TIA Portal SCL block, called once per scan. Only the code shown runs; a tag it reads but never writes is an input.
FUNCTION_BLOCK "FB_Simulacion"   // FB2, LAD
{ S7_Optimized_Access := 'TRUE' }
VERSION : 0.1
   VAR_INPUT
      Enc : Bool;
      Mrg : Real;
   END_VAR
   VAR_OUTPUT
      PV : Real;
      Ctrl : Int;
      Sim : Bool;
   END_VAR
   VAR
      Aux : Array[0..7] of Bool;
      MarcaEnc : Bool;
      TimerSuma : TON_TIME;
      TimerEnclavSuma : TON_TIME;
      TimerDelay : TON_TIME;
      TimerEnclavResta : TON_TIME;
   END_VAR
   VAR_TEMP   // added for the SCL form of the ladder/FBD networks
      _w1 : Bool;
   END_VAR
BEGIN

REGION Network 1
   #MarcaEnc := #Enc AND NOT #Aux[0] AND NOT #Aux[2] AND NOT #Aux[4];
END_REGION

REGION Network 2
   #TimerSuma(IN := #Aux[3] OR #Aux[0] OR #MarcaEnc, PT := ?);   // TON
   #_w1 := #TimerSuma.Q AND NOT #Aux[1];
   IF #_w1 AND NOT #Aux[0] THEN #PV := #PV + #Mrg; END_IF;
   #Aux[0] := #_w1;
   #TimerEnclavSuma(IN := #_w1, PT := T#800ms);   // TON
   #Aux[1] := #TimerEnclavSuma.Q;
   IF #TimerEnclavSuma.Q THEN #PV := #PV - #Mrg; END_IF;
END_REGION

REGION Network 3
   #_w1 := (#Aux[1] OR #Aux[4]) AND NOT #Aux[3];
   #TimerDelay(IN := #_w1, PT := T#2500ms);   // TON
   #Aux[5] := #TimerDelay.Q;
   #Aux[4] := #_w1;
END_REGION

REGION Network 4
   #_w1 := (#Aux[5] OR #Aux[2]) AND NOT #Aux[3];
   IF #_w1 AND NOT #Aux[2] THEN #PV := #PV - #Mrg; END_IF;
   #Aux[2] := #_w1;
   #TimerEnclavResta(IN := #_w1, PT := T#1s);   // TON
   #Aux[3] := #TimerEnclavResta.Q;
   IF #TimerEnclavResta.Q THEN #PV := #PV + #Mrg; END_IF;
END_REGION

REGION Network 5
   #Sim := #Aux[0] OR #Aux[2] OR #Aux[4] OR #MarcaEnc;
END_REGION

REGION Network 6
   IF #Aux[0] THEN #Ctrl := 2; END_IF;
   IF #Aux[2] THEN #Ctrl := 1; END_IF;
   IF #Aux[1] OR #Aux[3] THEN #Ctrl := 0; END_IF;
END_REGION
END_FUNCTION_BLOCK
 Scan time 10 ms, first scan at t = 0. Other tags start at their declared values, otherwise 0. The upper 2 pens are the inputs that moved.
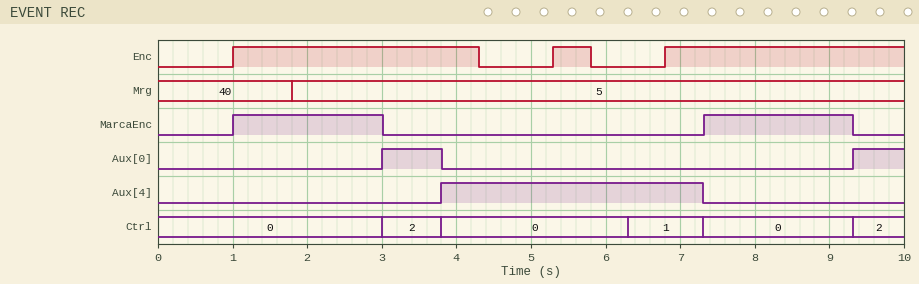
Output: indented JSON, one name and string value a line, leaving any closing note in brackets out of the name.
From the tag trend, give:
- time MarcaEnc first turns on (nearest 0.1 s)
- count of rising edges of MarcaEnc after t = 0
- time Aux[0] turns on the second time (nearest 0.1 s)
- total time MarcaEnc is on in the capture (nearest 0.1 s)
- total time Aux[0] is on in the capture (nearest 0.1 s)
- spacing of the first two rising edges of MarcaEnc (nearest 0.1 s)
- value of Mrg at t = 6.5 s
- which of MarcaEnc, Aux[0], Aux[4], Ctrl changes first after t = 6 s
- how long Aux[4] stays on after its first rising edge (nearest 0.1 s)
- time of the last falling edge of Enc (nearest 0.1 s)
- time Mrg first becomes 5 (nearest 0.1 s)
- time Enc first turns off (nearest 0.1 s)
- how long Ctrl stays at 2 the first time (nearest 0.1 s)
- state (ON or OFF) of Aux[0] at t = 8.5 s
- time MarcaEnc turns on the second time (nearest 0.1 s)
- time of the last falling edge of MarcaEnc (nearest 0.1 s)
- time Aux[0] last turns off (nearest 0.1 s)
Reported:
{
  "time MarcaEnc first turns on": "1.0 s",
  "count of rising edges of MarcaEnc after t = 0": "2",
  "time Aux[0] turns on the second time": "9.3 s",
  "total time MarcaEnc is on in the capture": "4.0 s",
  "total time Aux[0] is on in the capture": "1.5 s",
  "spacing of the first two rising edges of MarcaEnc": "6.3 s",
  "value of Mrg at t = 6.5 s": "5",
  "which of MarcaEnc, Aux[0], Aux[4], Ctrl changes first after t = 6 s": "Ctrl",
  "how long Aux[4] stays on after its first rising edge": "3.5 s",
  "time of the last falling edge of Enc": "5.8 s",
  "time Mrg first becomes 5": "1.8 s",
  "time Enc first turns off": "4.3 s",
  "how long Ctrl stays at 2 the first time": "0.8 s",
  "state (ON or OFF) of Aux[0] at t = 8.5 s": "OFF",
  "time MarcaEnc turns on the second time": "7.3 s",
  "time of the last falling edge of MarcaEnc": "9.3 s",
  "time Aux[0] last turns off": "3.8 s"
}
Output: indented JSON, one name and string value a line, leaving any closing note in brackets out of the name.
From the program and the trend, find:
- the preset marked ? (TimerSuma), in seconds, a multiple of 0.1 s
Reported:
{
  "the preset marked ? (TimerSuma), in seconds, a multiple of 0.1 s": "2.0 s"
}
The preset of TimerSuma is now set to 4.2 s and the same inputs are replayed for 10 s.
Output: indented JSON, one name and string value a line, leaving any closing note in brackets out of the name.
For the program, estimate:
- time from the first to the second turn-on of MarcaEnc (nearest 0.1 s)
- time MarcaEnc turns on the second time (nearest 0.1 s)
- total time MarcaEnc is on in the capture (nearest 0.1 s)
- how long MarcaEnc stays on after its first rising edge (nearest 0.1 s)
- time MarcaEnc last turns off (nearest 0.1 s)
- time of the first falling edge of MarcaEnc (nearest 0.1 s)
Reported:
{
  "time from the first to the second turn-on of MarcaEnc": "4.3 s",
  "time MarcaEnc turns on the second time": "5.3 s",
  "total time MarcaEnc is on in the capture": "7.0 s",
  "how long MarcaEnc stays on after its first rising edge": "3.3 s",
  "time MarcaEnc last turns off": "5.8 s",
  "time of the first falling edge of MarcaEnc": "4.3 s"
}
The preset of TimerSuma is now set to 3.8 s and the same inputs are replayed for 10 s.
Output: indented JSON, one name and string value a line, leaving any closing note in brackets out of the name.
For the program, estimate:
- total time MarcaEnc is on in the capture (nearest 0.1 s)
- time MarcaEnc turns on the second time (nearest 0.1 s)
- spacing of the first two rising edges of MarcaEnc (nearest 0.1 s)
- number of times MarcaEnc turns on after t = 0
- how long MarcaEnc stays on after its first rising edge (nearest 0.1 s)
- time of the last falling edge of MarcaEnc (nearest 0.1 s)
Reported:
{
  "total time MarcaEnc is on in the capture": "7.0 s",
  "time MarcaEnc turns on the second time": "5.3 s",
  "spacing of the first two rising edges of MarcaEnc": "4.3 s",
  "number of times MarcaEnc turns on after t = 0": "3",
  "how long MarcaEnc stays on after its first rising edge": "3.3 s",
  "time of the last falling edge of MarcaEnc": "5.8 s"
}
